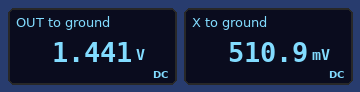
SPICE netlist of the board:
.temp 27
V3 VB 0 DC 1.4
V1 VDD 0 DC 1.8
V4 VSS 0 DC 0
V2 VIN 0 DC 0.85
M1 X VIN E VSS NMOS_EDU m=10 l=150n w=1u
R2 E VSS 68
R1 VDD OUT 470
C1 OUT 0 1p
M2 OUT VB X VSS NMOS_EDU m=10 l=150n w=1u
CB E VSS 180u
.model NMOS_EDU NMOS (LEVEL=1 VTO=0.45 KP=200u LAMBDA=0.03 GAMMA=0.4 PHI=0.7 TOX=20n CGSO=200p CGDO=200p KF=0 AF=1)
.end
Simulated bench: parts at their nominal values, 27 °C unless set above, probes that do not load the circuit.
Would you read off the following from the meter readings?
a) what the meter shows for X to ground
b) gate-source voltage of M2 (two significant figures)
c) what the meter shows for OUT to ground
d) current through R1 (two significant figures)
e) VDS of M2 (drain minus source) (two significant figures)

510.9 mV
890 mV
1.441 V
760 µA
930 mV
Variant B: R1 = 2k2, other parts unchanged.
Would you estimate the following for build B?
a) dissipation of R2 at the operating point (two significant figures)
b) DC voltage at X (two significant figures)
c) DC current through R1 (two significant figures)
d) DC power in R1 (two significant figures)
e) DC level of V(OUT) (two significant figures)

30 µW
250 mV
670 µA
980 µW
330 mV
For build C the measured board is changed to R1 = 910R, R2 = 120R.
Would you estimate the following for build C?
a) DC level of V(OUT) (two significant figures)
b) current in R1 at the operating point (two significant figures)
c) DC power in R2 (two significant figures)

1.2 V
630 µA
48 µW
